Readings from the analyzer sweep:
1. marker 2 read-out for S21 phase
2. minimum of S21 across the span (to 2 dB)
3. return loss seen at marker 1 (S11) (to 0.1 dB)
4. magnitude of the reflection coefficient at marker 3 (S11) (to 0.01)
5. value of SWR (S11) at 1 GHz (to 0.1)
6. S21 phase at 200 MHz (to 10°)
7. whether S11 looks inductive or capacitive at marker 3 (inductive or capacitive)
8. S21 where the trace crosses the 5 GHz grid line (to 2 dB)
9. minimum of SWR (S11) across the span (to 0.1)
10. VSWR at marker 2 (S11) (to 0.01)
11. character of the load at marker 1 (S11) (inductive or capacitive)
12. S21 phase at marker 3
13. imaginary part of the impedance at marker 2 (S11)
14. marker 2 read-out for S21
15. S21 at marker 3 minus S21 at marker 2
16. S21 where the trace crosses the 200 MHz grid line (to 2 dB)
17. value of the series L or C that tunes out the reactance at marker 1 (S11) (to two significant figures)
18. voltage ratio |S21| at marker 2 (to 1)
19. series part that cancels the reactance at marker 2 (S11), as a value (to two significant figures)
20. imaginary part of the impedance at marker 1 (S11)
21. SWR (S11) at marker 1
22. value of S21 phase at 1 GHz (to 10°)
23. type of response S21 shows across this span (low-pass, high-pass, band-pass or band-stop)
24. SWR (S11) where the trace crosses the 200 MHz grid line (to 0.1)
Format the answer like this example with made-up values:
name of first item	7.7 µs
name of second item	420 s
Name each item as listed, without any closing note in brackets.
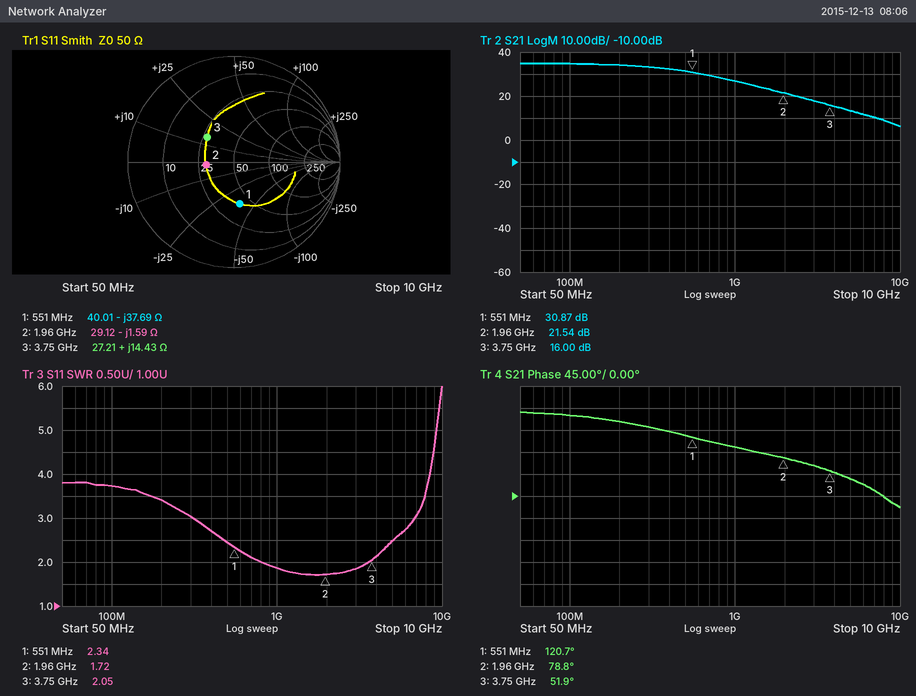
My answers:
marker 2 read-out for S21 phase	78.8°
minimum of S21 across the span	6 dB
return loss seen at marker 1 (S11)	8.0 dB
magnitude of the reflection coefficient at marker 3 (S11)	0.34
value of SWR (S11) at 1 GHz	1.9
S21 phase at 200 MHz	150°
whether S11 looks inductive or capacitive at marker 3	inductive
S21 where the trace crosses the 5 GHz grid line	14 dB
minimum of SWR (S11) across the span	1.7
VSWR at marker 2 (S11)	1.72
character of the load at marker 1 (S11)	capacitive
S21 phase at marker 3	51.9°
imaginary part of the impedance at marker 2	-1.59 Ω
marker 2 read-out for S21	21.54 dB
S21 at marker 3 minus S21 at marker 2	-5.54 dB
S21 where the trace crosses the 200 MHz grid line	34 dB
value of the series L or C that tunes out the reactance at marker 1 (S11)	11 nH
voltage ratio |S21| at marker 2	12
series part that cancels the reactance at marker 2 (S11), as a value	130 pH
imaginary part of the impedance at marker 1	-37.69 Ω
SWR (S11) at marker 1	2.34
value of S21 phase at 1 GHz	100°
type of response S21 shows across this span	low-pass
SWR (S11) where the trace crosses the 200 MHz grid line	3.4
